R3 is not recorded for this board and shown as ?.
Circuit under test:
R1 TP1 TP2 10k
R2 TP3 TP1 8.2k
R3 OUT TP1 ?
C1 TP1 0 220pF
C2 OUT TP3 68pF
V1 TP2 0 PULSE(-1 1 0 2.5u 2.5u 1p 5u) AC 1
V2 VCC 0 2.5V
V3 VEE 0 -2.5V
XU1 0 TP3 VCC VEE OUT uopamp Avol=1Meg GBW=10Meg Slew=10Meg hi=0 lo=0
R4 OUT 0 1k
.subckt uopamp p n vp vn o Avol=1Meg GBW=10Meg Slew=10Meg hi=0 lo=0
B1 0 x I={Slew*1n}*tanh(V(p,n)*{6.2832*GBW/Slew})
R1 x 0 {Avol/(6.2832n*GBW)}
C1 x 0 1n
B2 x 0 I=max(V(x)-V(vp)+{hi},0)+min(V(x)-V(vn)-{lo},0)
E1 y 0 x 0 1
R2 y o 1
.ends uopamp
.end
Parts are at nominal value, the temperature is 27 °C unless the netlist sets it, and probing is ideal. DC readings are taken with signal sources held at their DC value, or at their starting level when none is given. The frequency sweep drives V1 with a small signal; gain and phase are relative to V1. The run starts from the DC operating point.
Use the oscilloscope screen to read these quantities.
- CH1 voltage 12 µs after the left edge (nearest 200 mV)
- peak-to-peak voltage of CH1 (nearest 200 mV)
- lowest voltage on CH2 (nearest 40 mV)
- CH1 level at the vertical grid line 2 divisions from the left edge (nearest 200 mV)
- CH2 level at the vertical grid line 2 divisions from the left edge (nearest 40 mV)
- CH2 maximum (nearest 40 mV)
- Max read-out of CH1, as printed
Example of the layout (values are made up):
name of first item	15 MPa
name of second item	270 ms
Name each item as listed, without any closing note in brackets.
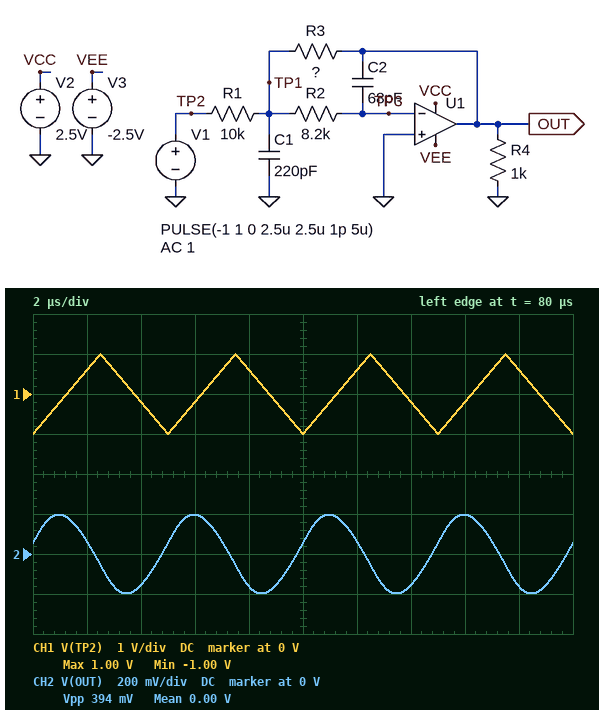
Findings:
CH1 voltage 12 µs after the left edge	600 mV
peak-to-peak voltage of CH1	2.0 V
lowest voltage on CH2	-200 mV
CH1 level at the vertical grid line 2 divisions from the left edge	-200 mV
CH2 level at the vertical grid line 2 divisions from the left edge	-160 mV
CH2 maximum	200 mV
Max read-out of CH1, as printed	1.00 V
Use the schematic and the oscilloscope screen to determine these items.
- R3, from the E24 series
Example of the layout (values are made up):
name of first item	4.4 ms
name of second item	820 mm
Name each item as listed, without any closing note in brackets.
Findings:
R3, from the E24 series	3 kΩ
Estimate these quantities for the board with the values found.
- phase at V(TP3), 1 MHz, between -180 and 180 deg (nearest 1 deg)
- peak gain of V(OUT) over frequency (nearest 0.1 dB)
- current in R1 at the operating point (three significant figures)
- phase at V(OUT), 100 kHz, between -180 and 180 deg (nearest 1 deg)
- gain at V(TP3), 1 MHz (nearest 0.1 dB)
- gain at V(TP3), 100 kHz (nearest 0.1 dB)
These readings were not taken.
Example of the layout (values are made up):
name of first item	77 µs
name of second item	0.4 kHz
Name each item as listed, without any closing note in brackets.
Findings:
phase at V(TP3), 1 MHz, between -180 and 180 deg	-73 deg
peak gain of V(OUT) over frequency	-10.5 dB
current in R1 at the operating point	100 µA
phase at V(OUT), 100 kHz, between -180 and 180 deg	145 deg
gain at V(TP3), 1 MHz	-54.1 dB
gain at V(TP3), 100 kHz	-50.7 dB
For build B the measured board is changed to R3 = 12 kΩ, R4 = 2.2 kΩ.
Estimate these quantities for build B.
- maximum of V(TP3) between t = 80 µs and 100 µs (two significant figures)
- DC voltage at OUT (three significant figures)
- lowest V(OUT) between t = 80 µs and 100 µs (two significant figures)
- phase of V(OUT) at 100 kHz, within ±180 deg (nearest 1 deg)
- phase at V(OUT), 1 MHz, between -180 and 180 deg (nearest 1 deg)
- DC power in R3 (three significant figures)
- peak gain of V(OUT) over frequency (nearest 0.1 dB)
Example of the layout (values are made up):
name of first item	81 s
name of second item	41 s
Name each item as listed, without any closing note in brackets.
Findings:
maximum of V(TP3) between t = 80 µs and 100 µs	6.9 mV
DC voltage at OUT	1.20 V
lowest V(OUT) between t = 80 µs and 100 µs	-330 mV
phase of V(OUT) at 100 kHz, within ±180 deg	107 deg
phase at V(OUT), 1 MHz, between -180 and 180 deg	7 deg
DC power in R3	120 µW
peak gain of V(OUT) over frequency	1.6 dB
